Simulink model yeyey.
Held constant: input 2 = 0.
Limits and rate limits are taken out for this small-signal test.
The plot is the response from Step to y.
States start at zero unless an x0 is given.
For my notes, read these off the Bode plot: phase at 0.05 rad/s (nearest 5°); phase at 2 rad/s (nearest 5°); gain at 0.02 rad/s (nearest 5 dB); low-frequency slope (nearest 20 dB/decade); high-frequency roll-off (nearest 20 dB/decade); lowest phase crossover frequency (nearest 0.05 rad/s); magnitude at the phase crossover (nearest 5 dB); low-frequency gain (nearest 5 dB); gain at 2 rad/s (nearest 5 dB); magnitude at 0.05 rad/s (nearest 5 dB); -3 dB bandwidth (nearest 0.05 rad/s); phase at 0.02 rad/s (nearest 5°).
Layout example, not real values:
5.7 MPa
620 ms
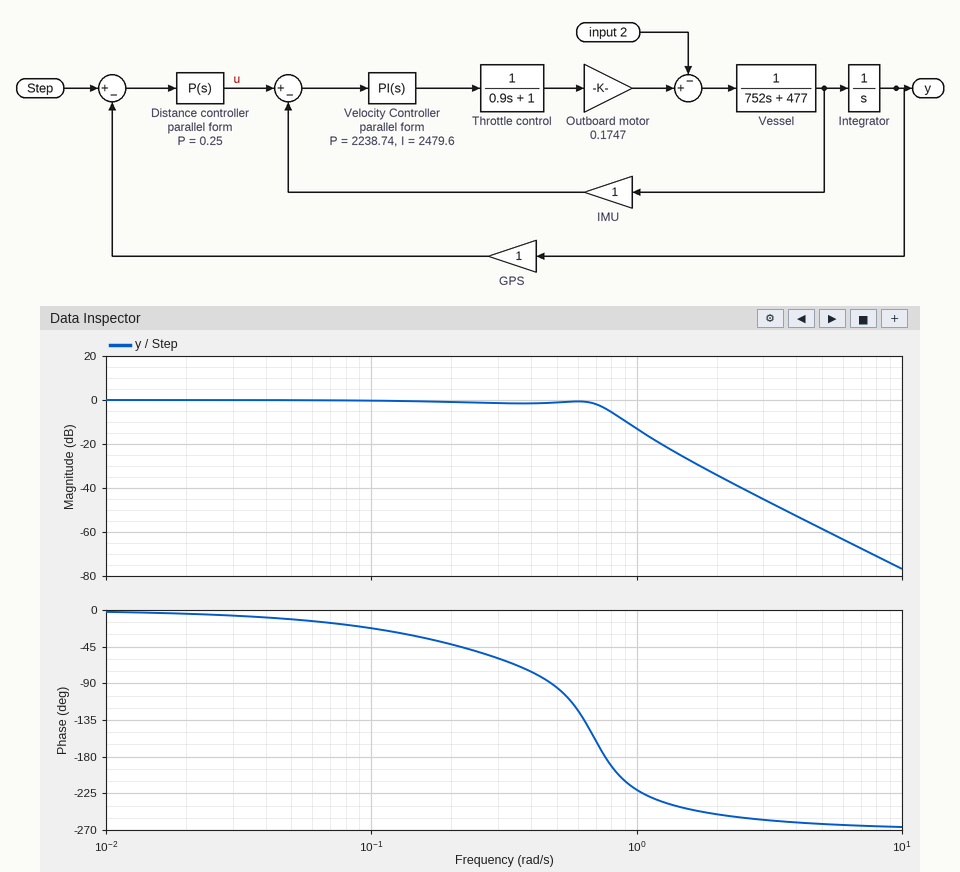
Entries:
-10°
-250°
0 dB
0 dB/decade
-60 dB/decade
0.75 rad/s
-5 dB
0 dB
-35 dB
0 dB
0.75 rad/s
-5°
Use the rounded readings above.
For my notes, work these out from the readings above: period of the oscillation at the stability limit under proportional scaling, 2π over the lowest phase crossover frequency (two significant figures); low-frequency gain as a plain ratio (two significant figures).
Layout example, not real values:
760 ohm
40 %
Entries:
8.4 s
1.0
